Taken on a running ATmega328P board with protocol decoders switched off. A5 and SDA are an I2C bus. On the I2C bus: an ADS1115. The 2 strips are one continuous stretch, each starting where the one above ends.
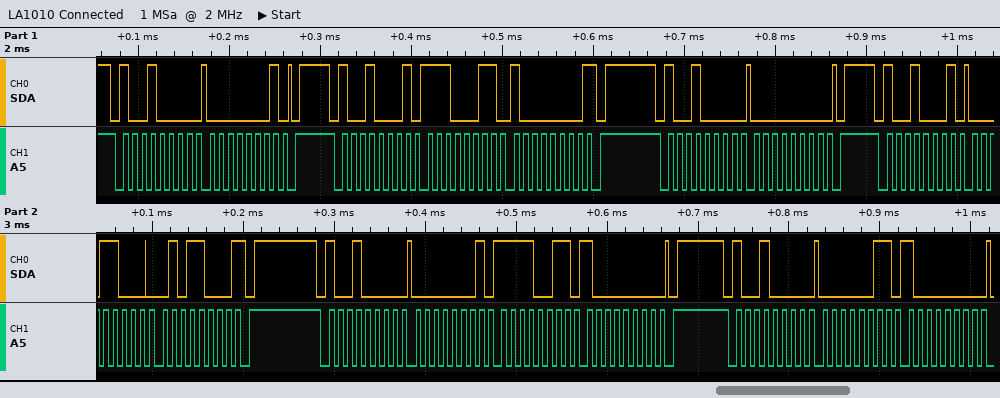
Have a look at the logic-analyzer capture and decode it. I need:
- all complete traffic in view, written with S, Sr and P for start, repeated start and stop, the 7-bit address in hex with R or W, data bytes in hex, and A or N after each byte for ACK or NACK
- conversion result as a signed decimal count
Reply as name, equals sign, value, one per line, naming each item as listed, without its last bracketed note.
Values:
all complete traffic in view, written with S, Sr and P for start, repeated start and stop, the 7-bit address in hex with R or W, data bytes in hex, and A or N after each byte for ACK or NACK = S 48W A 01 A P S 48R A E3 A 80 N P S 48W A 00 A P S 48R A 18 A 58 N P S 48W A 01 A F3 A 80 A P S 48W A 03 A 80 A
conversion result as a signed decimal count = 6232
